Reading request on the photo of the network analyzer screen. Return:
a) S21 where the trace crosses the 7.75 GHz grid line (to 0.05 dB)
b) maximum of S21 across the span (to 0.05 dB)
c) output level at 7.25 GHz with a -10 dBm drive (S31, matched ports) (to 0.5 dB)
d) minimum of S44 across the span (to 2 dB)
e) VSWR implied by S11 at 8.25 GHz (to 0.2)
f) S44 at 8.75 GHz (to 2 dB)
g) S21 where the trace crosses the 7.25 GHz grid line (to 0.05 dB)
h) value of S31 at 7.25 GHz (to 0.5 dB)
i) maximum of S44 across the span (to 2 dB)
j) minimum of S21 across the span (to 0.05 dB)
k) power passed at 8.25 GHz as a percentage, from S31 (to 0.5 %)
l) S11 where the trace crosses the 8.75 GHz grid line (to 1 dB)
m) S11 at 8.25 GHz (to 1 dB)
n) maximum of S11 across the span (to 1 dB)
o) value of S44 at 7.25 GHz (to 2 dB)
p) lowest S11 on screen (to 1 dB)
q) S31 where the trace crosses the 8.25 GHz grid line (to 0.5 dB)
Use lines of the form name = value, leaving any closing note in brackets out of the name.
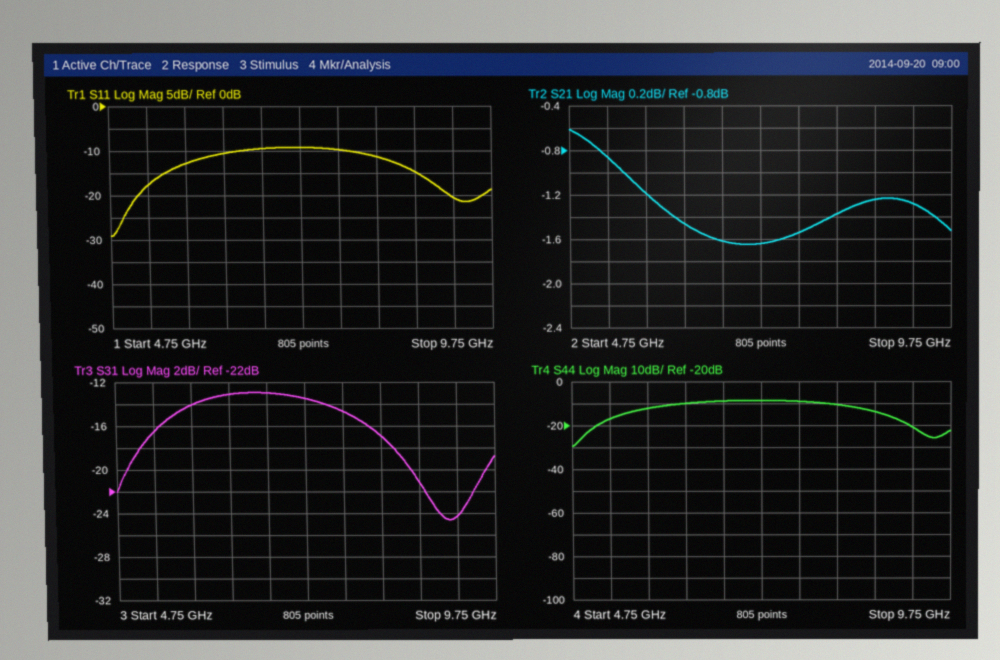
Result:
S21 where the trace crosses the 7.75 GHz grid line = -1.55 dB
maximum of S21 across the span = -0.60 dB
output level at 7.25 GHz with a -10 dBm drive (S31, matched ports) = -23.5 dBm
minimum of S44 across the span = -30 dB
VSWR implied by S11 at 8.25 GHz = 1.8
S44 at 8.75 GHz = -14 dB
S21 where the trace crosses the 7.25 GHz grid line = -1.65 dB
value of S31 at 7.25 GHz = -13.5 dB
maximum of S44 across the span = -8 dB
minimum of S21 across the span = -1.65 dB
power passed at 8.25 GHz as a percentage, from S31 = 2.0 %
S11 where the trace crosses the 8.75 GHz grid line = -15 dB
S11 at 8.25 GHz = -11 dB
maximum of S11 across the span = -9 dB
value of S44 at 7.25 GHz = -8 dB
lowest S11 on screen = -29 dB
S31 where the trace crosses the 8.25 GHz grid line = -17.0 dB
